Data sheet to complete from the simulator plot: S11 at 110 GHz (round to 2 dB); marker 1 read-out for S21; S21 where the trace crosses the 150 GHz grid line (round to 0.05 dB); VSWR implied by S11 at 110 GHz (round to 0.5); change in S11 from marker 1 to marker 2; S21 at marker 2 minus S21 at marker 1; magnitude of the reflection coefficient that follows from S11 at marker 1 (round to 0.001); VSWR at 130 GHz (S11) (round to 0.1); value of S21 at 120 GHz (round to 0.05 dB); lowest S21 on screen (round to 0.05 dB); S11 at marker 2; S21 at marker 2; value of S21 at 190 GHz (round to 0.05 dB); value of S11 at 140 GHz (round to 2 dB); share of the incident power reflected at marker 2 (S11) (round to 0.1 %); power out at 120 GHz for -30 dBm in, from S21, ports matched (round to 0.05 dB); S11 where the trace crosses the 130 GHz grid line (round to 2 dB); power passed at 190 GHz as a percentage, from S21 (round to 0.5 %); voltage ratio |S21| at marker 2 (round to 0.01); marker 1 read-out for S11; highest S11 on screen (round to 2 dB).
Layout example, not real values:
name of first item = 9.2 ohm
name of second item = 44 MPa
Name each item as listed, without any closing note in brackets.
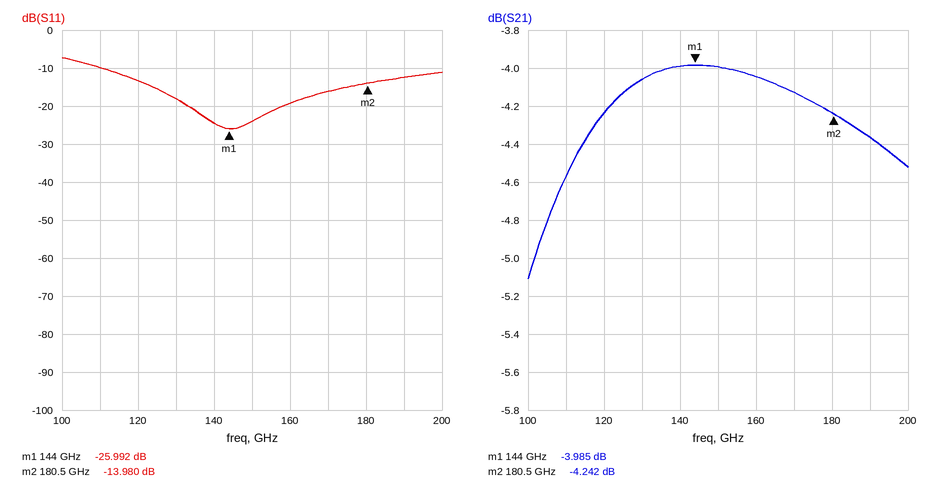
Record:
S11 at 110 GHz = -10 dB
marker 1 read-out for S21 = -3.985 dB
S21 where the trace crosses the 150 GHz grid line = -4.00 dB
VSWR implied by S11 at 110 GHz = 2.0
change in S11 from marker 1 to marker 2 = 12.012 dB
S21 at marker 2 minus S21 at marker 1 = -0.257 dB
magnitude of the reflection coefficient that follows from S11 at marker 1 = 0.050
VSWR at 130 GHz (S11) = 1.3
value of S21 at 120 GHz = -4.25 dB
lowest S21 on screen = -5.10 dB
S11 at marker 2 = -13.980 dB
S21 at marker 2 = -4.242 dB
value of S21 at 190 GHz = -4.35 dB
value of S11 at 140 GHz = -24 dB
share of the incident power reflected at marker 2 (S11) = 4.0 %
power out at 120 GHz for -30 dBm in, from S21, ports matched = -34.25 dBm
S11 where the trace crosses the 130 GHz grid line = -18 dB
power passed at 190 GHz as a percentage, from S21 = 36.5 %
voltage ratio |S21| at marker 2 = 0.61
marker 1 read-out for S11 = -25.992 dB
highest S11 on screen = -8 dB
